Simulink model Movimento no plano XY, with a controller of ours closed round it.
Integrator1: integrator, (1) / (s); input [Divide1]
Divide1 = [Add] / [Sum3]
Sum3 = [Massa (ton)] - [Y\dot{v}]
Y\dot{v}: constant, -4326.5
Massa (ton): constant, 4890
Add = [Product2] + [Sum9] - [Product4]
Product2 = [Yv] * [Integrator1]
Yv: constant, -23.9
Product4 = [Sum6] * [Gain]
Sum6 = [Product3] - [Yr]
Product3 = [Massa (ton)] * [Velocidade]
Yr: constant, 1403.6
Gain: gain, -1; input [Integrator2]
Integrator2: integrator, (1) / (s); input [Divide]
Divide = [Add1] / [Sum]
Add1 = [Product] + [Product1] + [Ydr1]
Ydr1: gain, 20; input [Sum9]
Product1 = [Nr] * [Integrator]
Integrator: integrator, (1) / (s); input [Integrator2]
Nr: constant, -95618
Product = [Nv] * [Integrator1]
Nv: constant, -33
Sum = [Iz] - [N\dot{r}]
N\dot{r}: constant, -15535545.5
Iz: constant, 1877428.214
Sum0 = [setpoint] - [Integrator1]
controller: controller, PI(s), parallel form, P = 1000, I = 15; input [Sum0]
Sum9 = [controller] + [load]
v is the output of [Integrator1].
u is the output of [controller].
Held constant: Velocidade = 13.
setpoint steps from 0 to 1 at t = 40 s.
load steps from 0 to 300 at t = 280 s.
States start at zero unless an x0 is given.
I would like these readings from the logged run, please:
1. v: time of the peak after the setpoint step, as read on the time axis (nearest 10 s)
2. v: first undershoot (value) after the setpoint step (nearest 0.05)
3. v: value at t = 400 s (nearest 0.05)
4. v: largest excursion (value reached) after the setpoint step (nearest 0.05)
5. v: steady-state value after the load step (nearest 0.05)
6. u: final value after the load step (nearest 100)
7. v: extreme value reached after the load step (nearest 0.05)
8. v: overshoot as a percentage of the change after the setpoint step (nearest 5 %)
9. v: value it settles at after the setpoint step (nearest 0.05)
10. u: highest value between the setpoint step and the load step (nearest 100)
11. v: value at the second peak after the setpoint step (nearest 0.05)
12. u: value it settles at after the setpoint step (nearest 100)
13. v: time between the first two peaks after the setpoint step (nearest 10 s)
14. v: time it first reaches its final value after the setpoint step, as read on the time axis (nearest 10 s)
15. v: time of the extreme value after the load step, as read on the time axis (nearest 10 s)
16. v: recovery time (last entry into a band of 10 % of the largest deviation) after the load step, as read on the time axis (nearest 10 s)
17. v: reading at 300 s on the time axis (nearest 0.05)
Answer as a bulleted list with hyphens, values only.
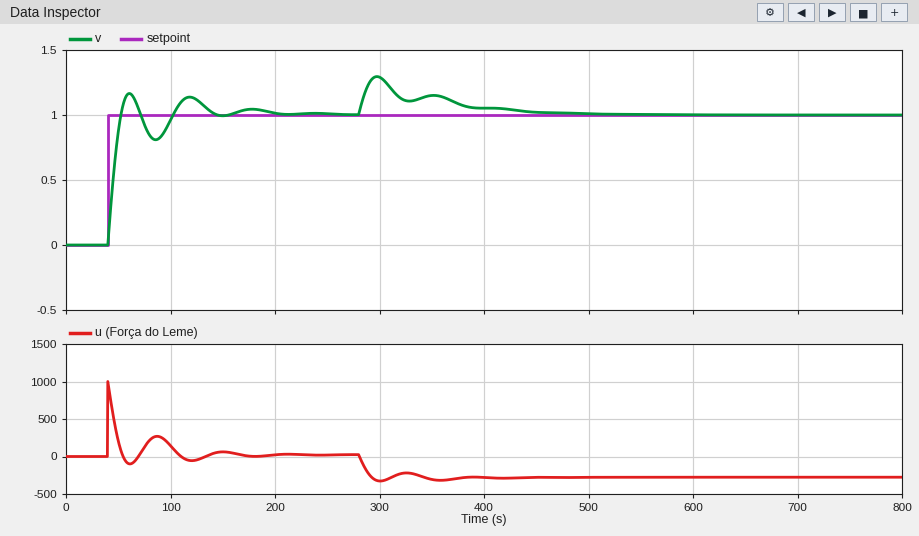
- 60 s
- 0.80
- 1.05
- 1.15
- 1.00
- -300
- 1.30
- 15 %
- 1.00
- 1000
- 1.15
- 0
- 60 s
- 50 s
- 300 s
- 440 s
- 1.30
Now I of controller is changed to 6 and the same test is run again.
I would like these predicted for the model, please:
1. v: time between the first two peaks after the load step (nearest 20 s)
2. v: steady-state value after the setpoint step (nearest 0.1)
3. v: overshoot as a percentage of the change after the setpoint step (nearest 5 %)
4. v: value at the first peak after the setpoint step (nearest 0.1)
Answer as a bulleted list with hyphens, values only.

- 60 s
- 1.0
- 10 %
- 1.1
